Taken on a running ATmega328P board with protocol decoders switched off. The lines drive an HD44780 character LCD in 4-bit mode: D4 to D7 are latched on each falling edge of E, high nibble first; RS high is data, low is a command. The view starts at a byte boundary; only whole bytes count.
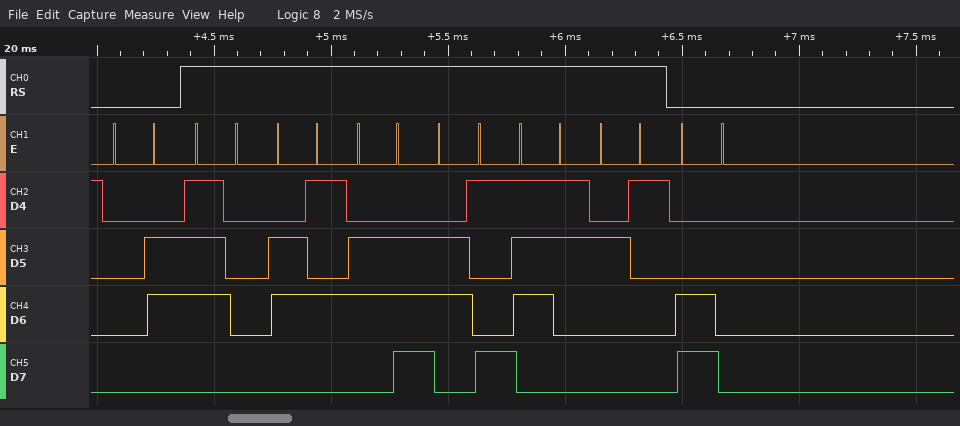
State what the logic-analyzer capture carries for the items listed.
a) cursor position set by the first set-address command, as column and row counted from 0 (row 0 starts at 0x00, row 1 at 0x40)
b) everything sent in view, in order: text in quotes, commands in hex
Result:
column 0, row 1
0x06 "penis!" 0xC0
